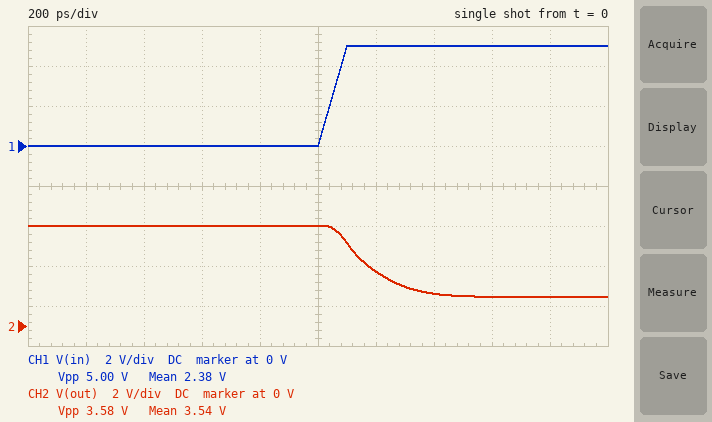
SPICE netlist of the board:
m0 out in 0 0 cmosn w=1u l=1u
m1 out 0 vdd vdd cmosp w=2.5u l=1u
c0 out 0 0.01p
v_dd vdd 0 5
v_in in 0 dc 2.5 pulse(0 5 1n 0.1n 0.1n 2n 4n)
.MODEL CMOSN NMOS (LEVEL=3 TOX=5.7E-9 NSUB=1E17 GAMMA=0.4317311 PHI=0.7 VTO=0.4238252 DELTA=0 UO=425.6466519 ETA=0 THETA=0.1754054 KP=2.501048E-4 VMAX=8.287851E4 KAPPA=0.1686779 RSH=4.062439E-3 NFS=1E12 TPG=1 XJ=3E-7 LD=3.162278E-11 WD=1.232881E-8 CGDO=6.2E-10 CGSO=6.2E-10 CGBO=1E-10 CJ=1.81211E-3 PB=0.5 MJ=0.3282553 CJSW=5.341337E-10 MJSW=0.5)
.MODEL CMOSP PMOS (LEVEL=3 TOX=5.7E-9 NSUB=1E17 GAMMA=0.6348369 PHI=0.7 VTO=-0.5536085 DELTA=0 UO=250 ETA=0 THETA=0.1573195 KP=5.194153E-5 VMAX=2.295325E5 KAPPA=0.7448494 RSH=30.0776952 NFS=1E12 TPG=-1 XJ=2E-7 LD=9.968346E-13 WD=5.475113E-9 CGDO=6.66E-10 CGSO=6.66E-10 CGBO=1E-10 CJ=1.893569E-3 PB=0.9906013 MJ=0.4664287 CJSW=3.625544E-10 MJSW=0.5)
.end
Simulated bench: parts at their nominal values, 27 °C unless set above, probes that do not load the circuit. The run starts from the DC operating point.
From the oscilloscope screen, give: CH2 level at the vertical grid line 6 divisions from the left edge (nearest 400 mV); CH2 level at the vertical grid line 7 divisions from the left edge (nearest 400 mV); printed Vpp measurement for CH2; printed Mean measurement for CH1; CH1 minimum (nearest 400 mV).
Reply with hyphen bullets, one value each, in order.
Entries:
- 2.8 V
- 1.6 V
- 3.58 V
- 2.38 V
- 0 V
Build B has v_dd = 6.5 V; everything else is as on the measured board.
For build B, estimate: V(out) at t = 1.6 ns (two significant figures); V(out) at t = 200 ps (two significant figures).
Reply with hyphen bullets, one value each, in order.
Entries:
- 4.0 V
- 6.5 V
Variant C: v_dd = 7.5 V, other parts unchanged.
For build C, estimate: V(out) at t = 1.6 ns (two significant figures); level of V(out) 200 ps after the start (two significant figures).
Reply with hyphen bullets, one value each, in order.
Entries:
- 5.4 V
- 7.5 V
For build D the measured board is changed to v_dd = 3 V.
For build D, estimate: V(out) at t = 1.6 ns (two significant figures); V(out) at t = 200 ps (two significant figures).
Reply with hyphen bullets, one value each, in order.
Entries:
- 400 mV
- 3.0 V
